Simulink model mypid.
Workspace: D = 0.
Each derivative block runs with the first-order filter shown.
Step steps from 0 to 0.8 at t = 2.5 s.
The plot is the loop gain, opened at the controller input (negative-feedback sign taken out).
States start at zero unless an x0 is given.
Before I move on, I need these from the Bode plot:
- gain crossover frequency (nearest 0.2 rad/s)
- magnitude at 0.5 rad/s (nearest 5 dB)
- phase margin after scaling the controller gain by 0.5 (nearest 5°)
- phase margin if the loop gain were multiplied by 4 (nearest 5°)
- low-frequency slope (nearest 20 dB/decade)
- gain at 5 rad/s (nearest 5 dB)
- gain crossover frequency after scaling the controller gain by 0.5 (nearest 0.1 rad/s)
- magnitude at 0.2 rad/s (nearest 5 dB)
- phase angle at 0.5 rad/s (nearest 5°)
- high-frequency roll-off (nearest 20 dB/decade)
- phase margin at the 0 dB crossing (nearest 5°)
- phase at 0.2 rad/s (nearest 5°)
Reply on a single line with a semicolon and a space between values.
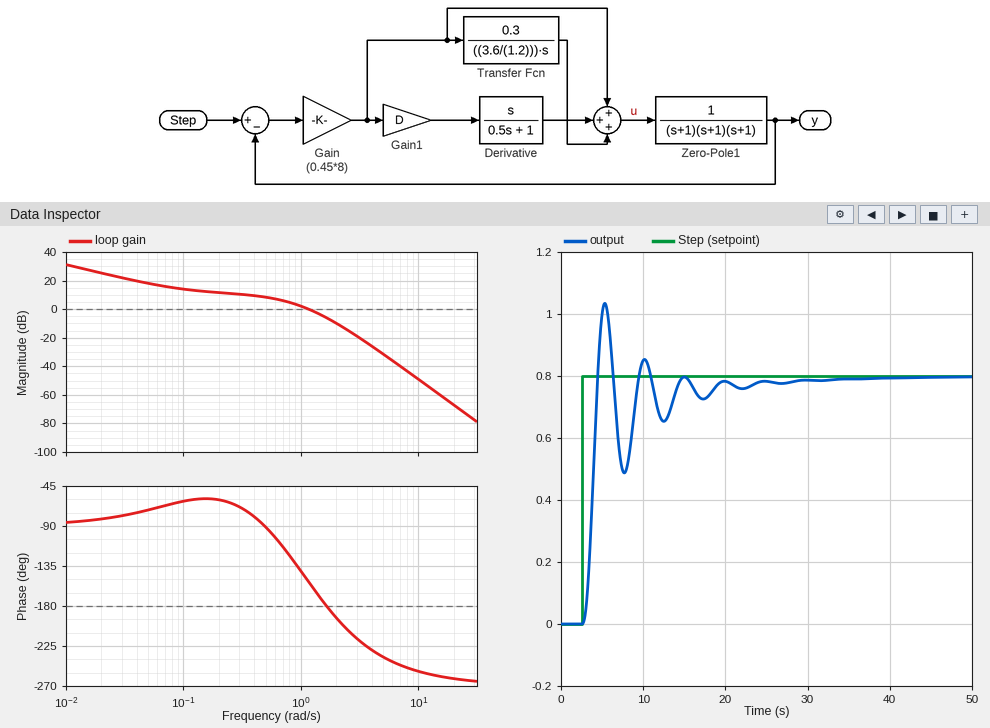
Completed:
1.2 rad/s; 10 dB; 65°; -20°; -20 dB/decade; -30 dB; 0.7 rad/s; 10 dB; -90°; -60 dB/decade; 25°; -60°
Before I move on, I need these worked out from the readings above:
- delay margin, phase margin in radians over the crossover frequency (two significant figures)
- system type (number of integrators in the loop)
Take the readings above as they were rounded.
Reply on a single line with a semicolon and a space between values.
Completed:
0.36 s; 1
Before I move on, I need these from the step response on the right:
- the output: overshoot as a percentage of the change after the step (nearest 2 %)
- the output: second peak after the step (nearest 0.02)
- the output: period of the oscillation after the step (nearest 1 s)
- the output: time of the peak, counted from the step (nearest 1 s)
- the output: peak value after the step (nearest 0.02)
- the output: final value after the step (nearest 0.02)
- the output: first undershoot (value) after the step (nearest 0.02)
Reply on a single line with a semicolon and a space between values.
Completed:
30 %; 0.86; 5 s; 3 s; 1.04; 0.80; 0.48
